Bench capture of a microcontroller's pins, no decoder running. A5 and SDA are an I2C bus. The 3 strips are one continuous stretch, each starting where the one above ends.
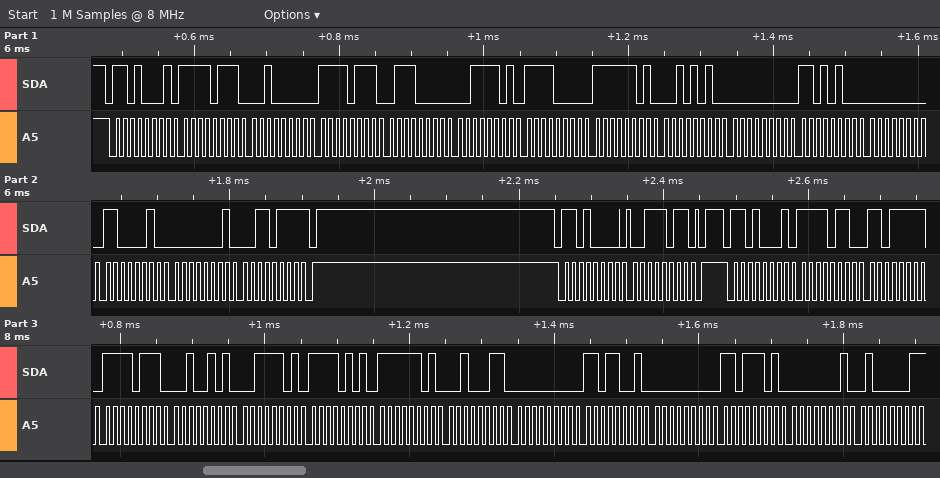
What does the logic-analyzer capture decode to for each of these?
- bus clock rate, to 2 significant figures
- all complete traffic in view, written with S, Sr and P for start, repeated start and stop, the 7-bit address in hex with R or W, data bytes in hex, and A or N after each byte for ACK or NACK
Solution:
100 kHz
S 68R A F7 A 20 A F7 A 70 A 3D A F0 A FD A 2A A 00 A D4 A 00 A C2 A 01 A 37 N P S 68W A 3B A P S 68R A F6 A DF A F7 A 25 A 3D A F5 A FD A 23 A 00 A D9 A 00 A DD A 01 A 41 N
